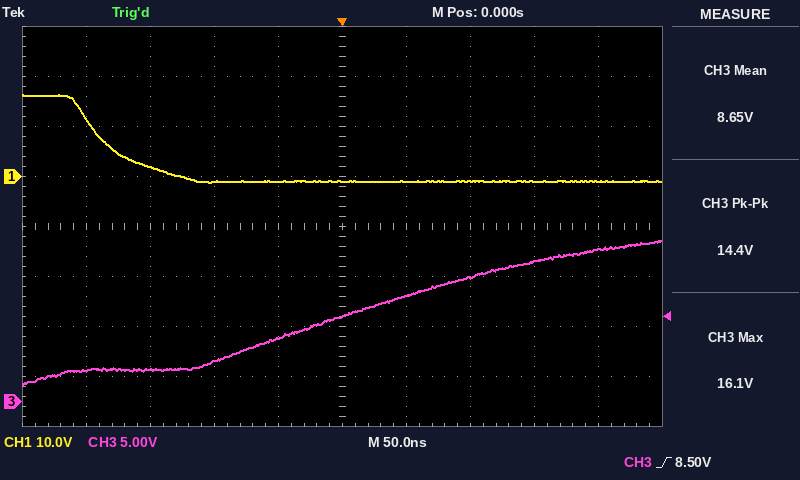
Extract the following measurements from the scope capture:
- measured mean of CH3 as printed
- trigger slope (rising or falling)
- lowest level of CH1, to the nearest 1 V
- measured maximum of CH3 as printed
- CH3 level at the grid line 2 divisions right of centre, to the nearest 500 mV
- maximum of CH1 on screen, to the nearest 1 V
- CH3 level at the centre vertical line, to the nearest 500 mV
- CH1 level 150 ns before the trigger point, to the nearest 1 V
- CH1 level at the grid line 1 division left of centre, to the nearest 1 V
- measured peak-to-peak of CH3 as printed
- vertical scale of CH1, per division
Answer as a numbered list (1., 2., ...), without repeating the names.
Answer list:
1. 8.65 V
2. rising
3. -1 V
4. 16.1 V
5. 12.5 V
6. 16 V
7. 8.5 V
8. 2 V
9. -1 V
10. 14.4 V
11. 10 V
